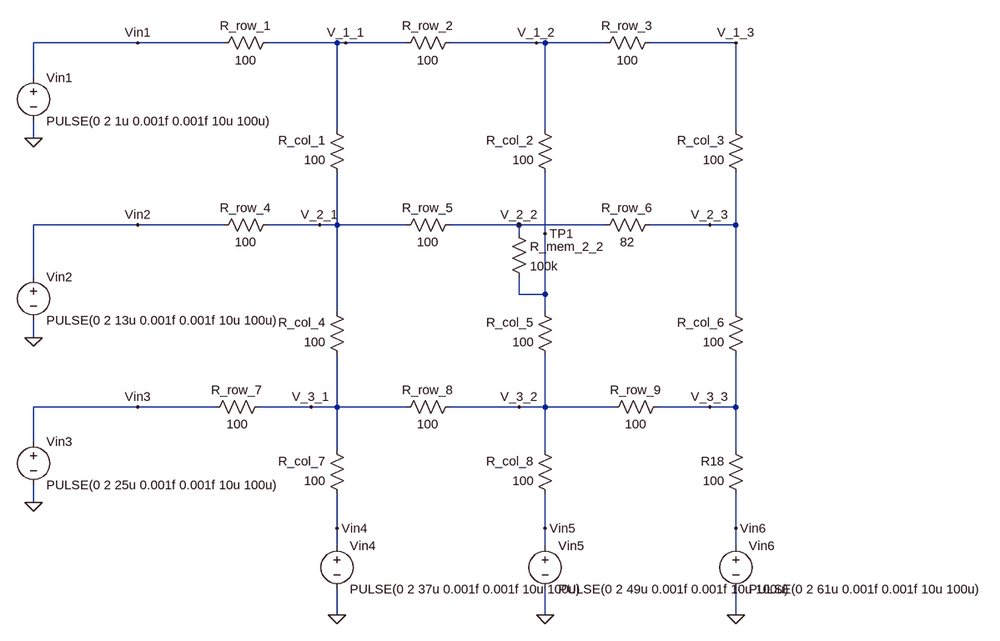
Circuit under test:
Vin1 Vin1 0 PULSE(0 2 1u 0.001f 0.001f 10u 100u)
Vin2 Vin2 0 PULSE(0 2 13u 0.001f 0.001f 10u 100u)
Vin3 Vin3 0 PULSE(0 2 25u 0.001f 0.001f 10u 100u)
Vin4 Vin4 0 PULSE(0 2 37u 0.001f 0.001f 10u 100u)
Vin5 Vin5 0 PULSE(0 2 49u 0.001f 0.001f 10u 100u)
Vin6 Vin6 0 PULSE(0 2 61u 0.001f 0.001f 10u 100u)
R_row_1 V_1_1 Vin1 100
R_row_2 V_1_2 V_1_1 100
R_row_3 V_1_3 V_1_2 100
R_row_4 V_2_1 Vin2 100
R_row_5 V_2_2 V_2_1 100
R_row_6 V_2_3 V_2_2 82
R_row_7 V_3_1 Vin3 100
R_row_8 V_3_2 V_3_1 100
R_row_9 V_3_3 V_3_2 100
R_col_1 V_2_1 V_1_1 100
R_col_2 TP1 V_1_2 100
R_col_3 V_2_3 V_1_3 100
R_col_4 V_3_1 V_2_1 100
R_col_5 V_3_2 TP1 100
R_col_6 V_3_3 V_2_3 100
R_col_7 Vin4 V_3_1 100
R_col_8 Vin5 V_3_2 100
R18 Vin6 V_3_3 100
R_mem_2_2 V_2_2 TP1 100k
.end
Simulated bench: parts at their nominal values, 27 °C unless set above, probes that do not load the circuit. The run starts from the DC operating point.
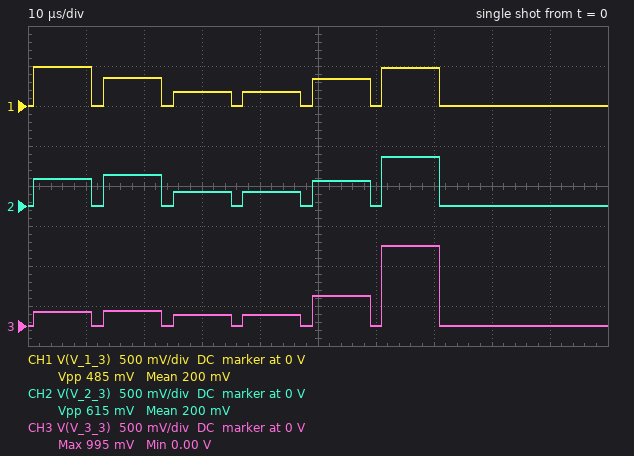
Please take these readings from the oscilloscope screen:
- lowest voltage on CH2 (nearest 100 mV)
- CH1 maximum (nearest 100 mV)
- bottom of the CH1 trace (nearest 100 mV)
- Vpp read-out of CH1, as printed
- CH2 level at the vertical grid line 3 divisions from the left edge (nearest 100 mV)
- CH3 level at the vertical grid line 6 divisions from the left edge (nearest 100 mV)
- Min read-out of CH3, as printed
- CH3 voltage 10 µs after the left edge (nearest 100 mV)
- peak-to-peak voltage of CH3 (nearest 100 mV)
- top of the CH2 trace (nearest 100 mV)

0 V
500 mV
0 V
485 mV
200 mV
0 V
0.00 V
200 mV
1.0 V
600 mV
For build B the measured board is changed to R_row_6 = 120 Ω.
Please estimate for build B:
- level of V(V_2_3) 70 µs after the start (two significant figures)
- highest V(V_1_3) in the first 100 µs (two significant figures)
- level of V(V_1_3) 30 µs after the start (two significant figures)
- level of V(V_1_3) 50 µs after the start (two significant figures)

640 mV
490 mV
170 mV
350 mV
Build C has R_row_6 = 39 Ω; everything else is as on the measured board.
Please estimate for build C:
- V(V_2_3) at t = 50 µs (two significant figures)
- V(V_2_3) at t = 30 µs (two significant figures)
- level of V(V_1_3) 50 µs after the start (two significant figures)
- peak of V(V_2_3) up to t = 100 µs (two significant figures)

300 mV
180 mV
330 mV
580 mV
